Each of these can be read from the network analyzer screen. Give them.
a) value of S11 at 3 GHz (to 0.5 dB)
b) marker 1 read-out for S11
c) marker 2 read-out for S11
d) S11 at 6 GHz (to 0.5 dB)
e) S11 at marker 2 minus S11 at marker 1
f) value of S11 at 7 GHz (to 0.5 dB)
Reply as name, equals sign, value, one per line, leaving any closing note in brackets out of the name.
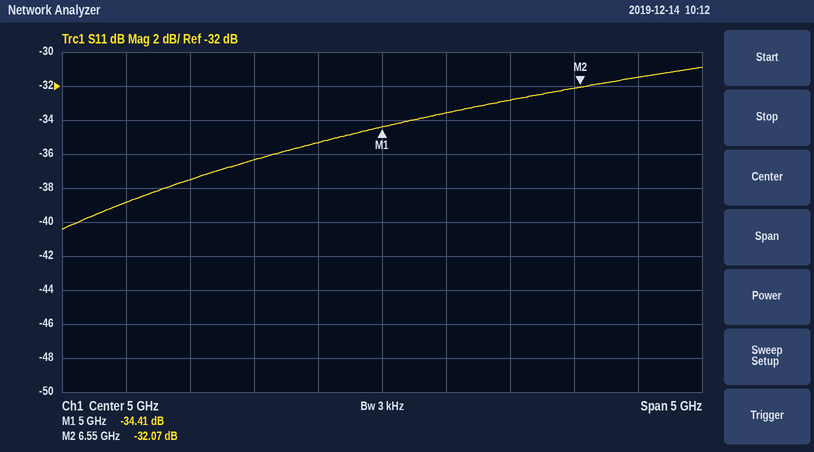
value of S11 at 3 GHz = -39.0 dB
marker 1 read-out for S11 = -34.41 dB
marker 2 read-out for S11 = -32.07 dB
S11 at 6 GHz = -33.0 dB
S11 at marker 2 minus S11 at marker 1 = 2.34 dB
value of S11 at 7 GHz = -31.5 dB
